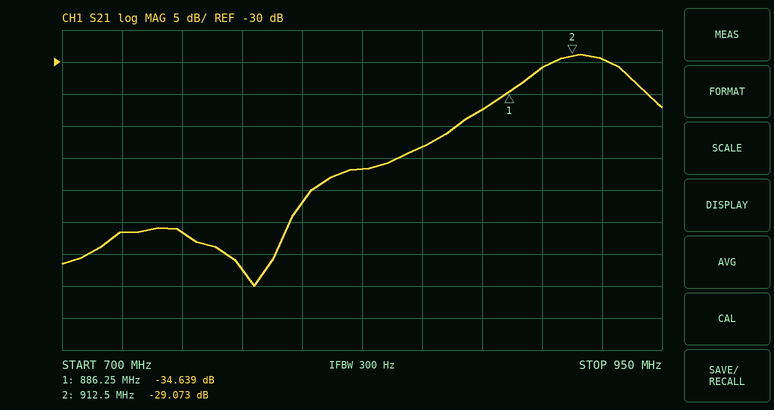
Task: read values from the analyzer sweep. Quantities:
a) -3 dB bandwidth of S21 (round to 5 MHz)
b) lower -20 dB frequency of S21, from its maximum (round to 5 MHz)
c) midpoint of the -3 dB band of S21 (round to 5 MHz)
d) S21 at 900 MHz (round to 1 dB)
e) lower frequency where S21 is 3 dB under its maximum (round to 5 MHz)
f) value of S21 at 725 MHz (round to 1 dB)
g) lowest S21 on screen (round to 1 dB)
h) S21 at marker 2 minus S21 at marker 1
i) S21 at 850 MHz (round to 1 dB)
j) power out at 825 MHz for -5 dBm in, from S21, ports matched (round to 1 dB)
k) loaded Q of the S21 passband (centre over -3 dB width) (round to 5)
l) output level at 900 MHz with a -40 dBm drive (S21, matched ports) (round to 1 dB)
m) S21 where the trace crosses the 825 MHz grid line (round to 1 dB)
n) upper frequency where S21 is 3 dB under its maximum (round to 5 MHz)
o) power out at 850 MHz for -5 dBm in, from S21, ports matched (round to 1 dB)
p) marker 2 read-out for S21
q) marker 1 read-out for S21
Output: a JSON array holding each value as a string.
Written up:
["40 MHz", "810 MHz", "915 MHz", "-31 dB", "895 MHz", "-57 dB", "-65 dB", "5.566 dB", "-43 dB", "-52 dBm", "25", "-71 dBm", "-47 dB", "935 MHz", "-48 dBm", "-29.073 dB", "-34.639 dB"]
